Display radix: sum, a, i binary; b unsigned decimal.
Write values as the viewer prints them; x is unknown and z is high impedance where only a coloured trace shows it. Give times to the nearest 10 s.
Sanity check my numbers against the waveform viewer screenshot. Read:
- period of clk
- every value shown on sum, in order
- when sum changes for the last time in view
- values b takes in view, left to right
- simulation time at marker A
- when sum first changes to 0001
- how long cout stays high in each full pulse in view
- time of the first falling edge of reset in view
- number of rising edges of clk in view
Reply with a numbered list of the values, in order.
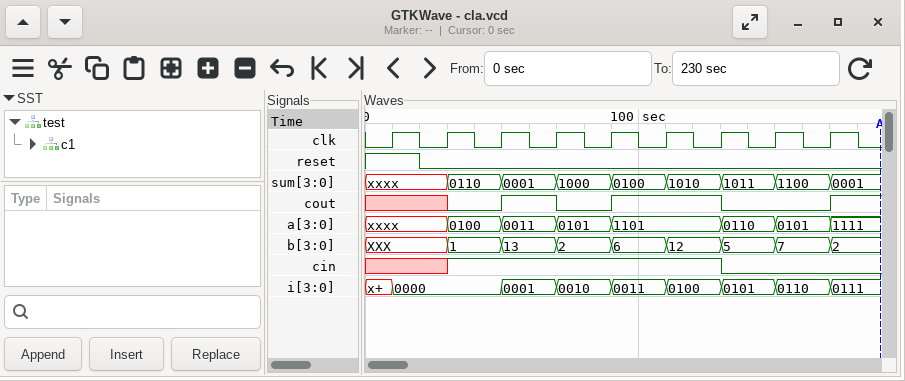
1. 20 s
2. xxxx, 0110, 0001, 1000, 0100, 1010, 1011, 1100, 0001
3. 170 s
4. XXX, 1, 13, 2, 6, 12, 5, 7, 2
5. 190 s
6. 50 s
7. 20 s, 40 s
8. 20 s
9. 9
